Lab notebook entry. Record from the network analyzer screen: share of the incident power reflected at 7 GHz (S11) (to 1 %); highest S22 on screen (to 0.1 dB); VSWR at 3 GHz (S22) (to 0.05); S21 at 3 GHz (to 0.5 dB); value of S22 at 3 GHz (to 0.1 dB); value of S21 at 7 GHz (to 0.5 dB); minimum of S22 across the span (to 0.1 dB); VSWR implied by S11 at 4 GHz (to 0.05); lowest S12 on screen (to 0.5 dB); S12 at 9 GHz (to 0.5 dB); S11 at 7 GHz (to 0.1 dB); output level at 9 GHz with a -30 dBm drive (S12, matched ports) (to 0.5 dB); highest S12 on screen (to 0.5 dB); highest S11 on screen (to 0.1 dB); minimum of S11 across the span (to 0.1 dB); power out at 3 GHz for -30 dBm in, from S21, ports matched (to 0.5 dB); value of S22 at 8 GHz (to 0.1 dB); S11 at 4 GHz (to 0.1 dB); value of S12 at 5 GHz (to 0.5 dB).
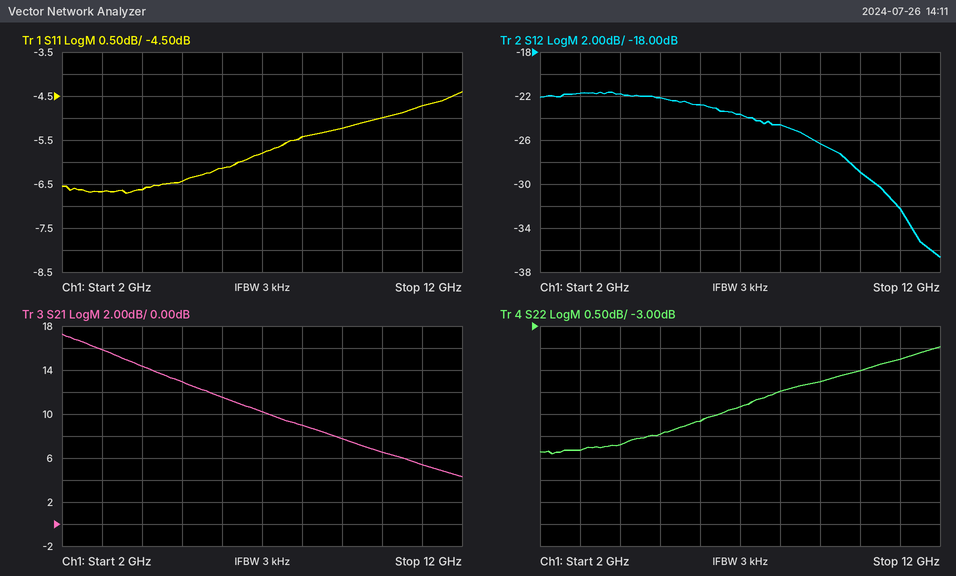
26 %
-3.5 dB
3.10
16.0 dB
-5.8 dB
10.0 dB
-5.9 dB
2.75
-36.5 dB
-26.5 dB
-5.8 dB
-56.5 dBm
-21.5 dB
-4.4 dB
-6.7 dB
-14.0 dBm
-4.5 dB
-6.6 dB
-22.0 dB
